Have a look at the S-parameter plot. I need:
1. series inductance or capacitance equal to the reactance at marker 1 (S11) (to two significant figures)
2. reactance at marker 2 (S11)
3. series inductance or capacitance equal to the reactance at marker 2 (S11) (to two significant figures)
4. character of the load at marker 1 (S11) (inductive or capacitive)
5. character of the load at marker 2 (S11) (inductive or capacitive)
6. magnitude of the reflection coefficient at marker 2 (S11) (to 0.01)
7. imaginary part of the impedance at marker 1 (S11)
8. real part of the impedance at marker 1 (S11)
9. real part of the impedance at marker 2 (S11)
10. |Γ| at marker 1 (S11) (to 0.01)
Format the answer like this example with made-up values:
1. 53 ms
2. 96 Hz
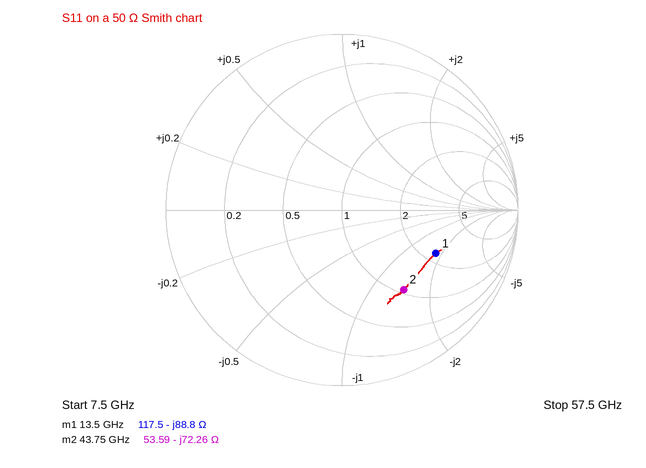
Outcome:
1. 130 fF
2. -72.26 Ω
3. 50 fF
4. capacitive
5. capacitive
6. 0.57
7. -88.8 Ω
8. 117.5 Ω
9. 53.59 Ω
10. 0.59
